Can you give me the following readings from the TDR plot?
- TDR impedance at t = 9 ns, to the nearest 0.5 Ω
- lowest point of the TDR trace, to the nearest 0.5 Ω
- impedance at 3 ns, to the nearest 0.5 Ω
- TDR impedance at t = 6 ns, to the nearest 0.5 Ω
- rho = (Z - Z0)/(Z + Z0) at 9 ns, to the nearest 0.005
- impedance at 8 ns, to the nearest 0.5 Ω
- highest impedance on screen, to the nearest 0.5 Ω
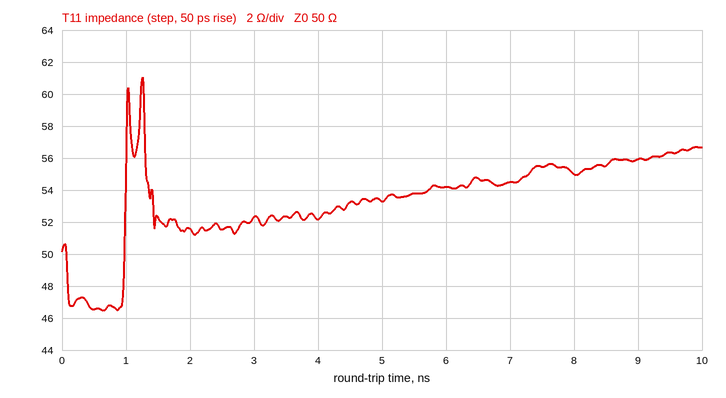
56.0 Ω
46.5 Ω
52.5 Ω
54.0 Ω
+0.055
55.0 Ω
61.0 Ω
